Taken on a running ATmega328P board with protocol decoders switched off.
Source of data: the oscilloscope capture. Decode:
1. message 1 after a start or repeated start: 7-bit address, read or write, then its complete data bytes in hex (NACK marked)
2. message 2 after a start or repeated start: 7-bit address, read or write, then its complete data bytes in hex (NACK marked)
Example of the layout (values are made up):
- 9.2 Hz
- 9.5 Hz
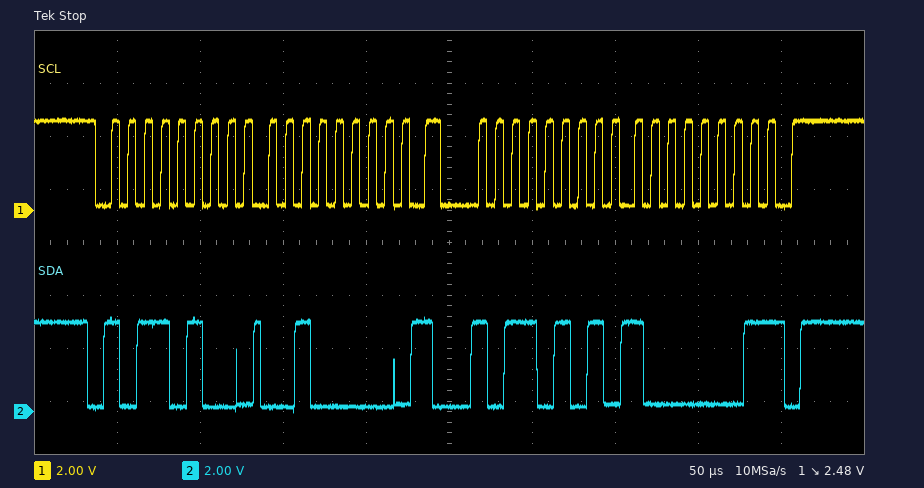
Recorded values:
- 0x5A write: 20
- 0x5A read: 81 NACK
